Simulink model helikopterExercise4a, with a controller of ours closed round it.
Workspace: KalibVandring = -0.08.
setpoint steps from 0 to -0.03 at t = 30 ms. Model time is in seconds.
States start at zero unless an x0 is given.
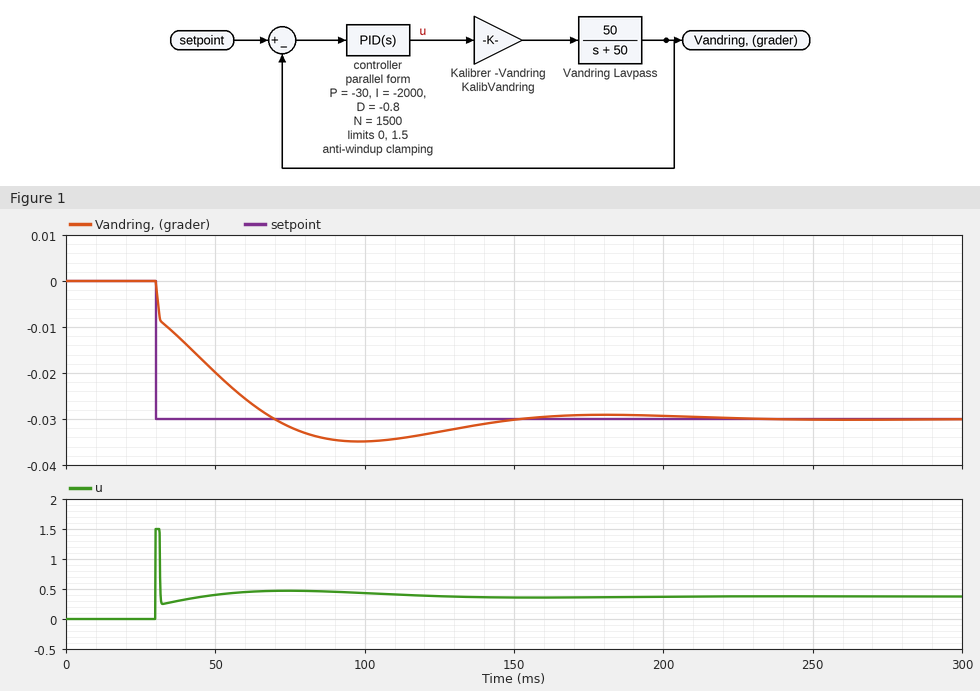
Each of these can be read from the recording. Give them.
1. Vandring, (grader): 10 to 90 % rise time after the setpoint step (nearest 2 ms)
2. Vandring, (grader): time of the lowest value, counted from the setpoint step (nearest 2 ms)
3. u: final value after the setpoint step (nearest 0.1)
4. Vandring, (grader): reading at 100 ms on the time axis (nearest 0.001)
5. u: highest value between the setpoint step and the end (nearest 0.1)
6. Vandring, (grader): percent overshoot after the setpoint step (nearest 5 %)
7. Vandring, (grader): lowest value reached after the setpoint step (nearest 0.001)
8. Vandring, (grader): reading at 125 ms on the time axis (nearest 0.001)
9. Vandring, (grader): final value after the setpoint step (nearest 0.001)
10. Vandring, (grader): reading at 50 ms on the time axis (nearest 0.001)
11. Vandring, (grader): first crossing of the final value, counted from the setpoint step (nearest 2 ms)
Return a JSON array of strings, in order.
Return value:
["32 ms", "68 ms", "0.4", "-0.035", "1.5", "15 %", "-0.035", "-0.033", "-0.030", "-0.020", "40 ms"]
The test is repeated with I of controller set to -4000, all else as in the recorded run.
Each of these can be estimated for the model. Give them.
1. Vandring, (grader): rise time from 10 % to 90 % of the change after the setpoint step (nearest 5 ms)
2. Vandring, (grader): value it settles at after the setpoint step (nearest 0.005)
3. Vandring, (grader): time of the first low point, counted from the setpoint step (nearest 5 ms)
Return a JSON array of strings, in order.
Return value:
["25 ms", "-0.030", "50 ms"]
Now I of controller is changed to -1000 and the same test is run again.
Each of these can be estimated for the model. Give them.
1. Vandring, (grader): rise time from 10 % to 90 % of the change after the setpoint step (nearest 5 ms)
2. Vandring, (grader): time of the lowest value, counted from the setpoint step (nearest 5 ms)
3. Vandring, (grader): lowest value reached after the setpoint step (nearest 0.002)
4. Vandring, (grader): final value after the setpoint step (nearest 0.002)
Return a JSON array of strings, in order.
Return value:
["45 ms", "100 ms", "-0.032", "-0.030"]
